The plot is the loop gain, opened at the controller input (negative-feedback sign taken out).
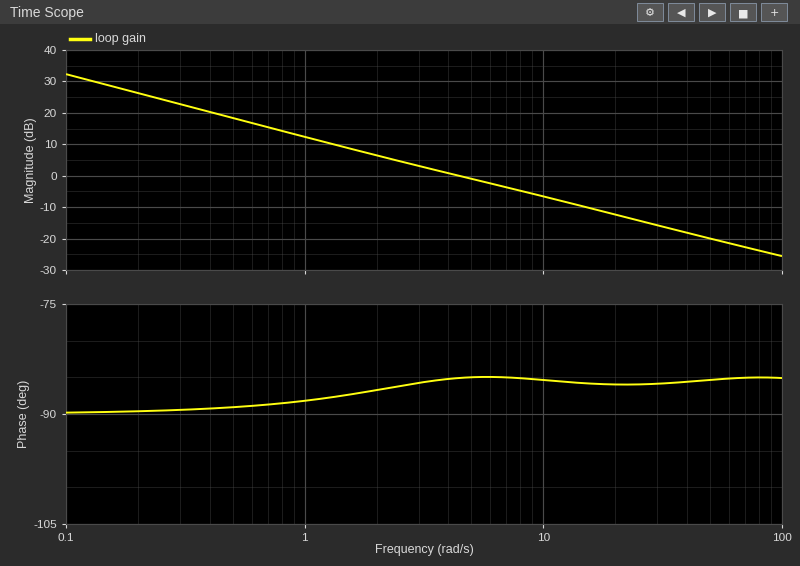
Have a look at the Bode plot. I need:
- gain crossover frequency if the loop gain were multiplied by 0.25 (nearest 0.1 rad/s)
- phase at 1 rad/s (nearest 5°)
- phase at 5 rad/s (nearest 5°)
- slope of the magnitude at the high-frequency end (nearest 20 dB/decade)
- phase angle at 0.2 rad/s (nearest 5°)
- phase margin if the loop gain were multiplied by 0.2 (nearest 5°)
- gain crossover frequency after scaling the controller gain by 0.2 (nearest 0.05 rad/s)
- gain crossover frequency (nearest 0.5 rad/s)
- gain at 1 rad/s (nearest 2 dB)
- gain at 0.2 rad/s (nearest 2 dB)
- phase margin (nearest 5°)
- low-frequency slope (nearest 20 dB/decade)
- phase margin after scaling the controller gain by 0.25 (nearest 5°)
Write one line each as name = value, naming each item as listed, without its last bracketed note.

gain crossover frequency if the loop gain were multiplied by 0.25 = 1.0 rad/s
phase at 1 rad/s = -90°
phase at 5 rad/s = -85°
slope of the magnitude at the high-frequency end = -20 dB/decade
phase angle at 0.2 rad/s = -90°
phase margin if the loop gain were multiplied by 0.2 = 90°
gain crossover frequency after scaling the controller gain by 0.2 = 0.85 rad/s
gain crossover frequency = 4.5 rad/s
gain at 1 rad/s = 12 dB
gain at 0.2 rad/s = 26 dB
phase margin = 95°
low-frequency slope = -20 dB/decade
phase margin after scaling the controller gain by 0.25 = 90°
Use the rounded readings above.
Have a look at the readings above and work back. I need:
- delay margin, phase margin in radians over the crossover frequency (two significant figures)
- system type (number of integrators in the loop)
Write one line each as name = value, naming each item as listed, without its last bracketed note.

delay margin, phase margin in radians over the crossover frequency = 0.37 s
system type = 1
